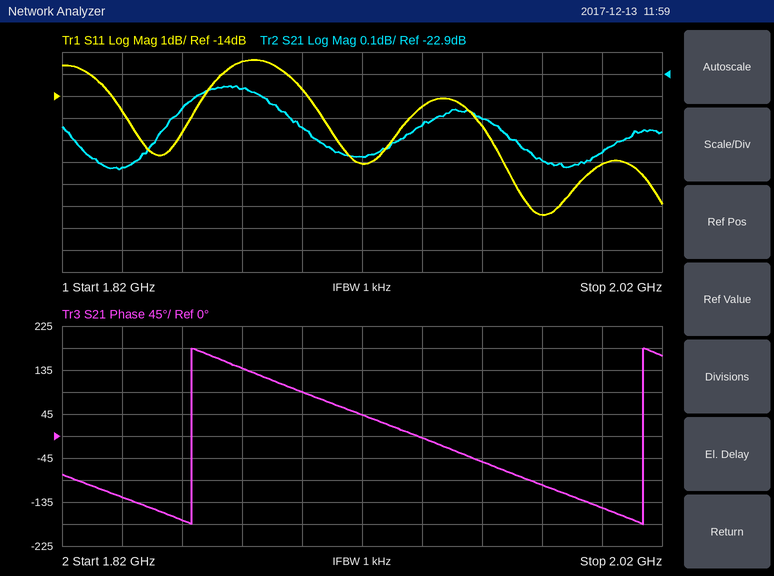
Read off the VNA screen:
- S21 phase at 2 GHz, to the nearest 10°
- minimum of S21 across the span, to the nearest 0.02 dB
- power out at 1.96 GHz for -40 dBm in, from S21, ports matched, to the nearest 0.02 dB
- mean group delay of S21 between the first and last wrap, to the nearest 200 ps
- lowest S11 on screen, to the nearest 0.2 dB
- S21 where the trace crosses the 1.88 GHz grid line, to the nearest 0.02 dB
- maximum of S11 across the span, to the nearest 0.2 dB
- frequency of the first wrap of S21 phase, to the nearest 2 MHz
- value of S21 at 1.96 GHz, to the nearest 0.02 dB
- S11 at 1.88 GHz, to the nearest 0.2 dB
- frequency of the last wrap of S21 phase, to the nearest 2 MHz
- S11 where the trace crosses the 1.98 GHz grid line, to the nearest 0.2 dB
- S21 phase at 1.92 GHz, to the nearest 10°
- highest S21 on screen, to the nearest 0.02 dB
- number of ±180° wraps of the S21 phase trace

-150°
-23.34 dB
-63.10 dBm
6.6 ns
-19.4 dB
-22.96 dB
-12.4 dB
1.864 GHz
-23.10 dB
-12.4 dB
2.014 GHz
-19.4 dB
40°
-22.96 dB
2
